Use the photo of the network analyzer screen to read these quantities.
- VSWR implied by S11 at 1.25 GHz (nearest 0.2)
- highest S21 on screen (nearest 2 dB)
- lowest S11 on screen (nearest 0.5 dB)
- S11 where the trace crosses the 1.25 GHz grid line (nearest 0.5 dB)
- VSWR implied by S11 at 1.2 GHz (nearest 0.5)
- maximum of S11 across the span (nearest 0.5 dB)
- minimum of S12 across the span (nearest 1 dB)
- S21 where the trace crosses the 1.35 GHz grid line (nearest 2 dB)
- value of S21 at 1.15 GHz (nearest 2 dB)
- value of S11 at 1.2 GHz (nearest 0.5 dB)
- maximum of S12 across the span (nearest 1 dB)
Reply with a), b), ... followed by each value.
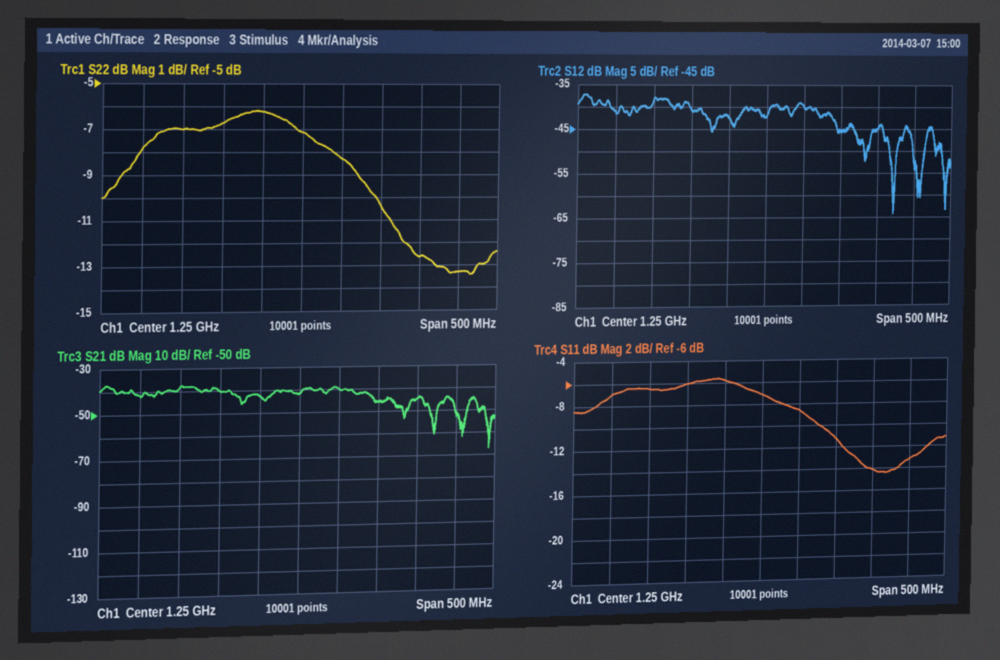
a) 2.6
b) -38 dB
c) -14.5 dB
d) -7.0 dB
e) 3.0
f) -5.5 dB
g) -64 dB
h) -46 dB
i) -40 dB
j) -6.0 dB
k) -37 dB
